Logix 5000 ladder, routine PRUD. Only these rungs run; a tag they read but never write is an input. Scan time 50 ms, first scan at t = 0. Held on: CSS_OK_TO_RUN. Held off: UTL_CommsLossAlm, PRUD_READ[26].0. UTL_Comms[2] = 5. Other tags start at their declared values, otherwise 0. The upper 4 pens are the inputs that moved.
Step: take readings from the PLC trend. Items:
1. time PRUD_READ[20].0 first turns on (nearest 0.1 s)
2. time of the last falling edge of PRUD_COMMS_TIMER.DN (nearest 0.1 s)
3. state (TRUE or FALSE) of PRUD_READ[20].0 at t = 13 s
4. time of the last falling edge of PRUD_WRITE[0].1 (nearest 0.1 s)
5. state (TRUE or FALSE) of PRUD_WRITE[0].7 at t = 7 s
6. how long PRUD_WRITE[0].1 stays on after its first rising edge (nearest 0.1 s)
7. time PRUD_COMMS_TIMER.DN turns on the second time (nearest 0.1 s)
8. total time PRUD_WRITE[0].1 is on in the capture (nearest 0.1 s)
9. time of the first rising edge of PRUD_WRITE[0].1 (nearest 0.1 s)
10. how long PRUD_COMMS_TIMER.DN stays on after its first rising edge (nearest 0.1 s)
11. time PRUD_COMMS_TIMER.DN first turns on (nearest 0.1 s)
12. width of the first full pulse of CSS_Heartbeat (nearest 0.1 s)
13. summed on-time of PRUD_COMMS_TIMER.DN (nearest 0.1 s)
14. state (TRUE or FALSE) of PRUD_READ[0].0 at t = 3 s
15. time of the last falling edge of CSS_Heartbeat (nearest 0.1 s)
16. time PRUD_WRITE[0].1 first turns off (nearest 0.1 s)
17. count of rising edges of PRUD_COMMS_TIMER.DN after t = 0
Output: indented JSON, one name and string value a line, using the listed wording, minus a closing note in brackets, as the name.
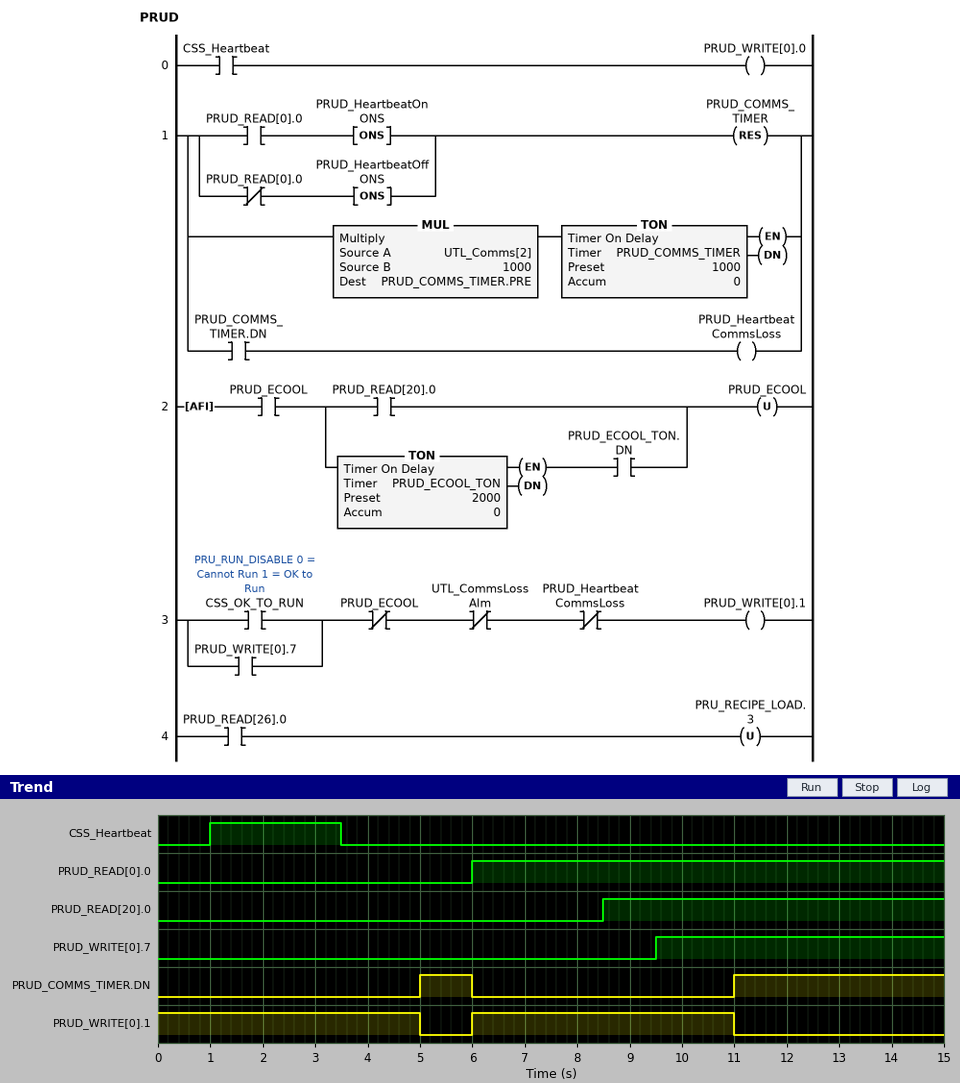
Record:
{
  "time PRUD_READ[20].0 first turns on": "8.5 s",
  "time of the last falling edge of PRUD_COMMS_TIMER.DN": "6.0 s",
  "state (TRUE or FALSE) of PRUD_READ[20].0 at t = 13 s": "TRUE",
  "time of the last falling edge of PRUD_WRITE[0].1": "11.0 s",
  "state (TRUE or FALSE) of PRUD_WRITE[0].7 at t = 7 s": "FALSE",
  "how long PRUD_WRITE[0].1 stays on after its first rising edge": "5.0 s",
  "time PRUD_COMMS_TIMER.DN turns on the second time": "11.0 s",
  "total time PRUD_WRITE[0].1 is on in the capture": "10.0 s",
  "time of the first rising edge of PRUD_WRITE[0].1": "6.0 s",
  "how long PRUD_COMMS_TIMER.DN stays on after its first rising edge": "1.0 s",
  "time PRUD_COMMS_TIMER.DN first turns on": "5.0 s",
  "width of the first full pulse of CSS_Heartbeat": "2.5 s",
  "summed on-time of PRUD_COMMS_TIMER.DN": "5.0 s",
  "state (TRUE or FALSE) of PRUD_READ[0].0 at t = 3 s": "FALSE",
  "time of the last falling edge of CSS_Heartbeat": "3.5 s",
  "time PRUD_WRITE[0].1 first turns off": "5.0 s",
  "count of rising edges of PRUD_COMMS_TIMER.DN after t = 0": "2"
}
